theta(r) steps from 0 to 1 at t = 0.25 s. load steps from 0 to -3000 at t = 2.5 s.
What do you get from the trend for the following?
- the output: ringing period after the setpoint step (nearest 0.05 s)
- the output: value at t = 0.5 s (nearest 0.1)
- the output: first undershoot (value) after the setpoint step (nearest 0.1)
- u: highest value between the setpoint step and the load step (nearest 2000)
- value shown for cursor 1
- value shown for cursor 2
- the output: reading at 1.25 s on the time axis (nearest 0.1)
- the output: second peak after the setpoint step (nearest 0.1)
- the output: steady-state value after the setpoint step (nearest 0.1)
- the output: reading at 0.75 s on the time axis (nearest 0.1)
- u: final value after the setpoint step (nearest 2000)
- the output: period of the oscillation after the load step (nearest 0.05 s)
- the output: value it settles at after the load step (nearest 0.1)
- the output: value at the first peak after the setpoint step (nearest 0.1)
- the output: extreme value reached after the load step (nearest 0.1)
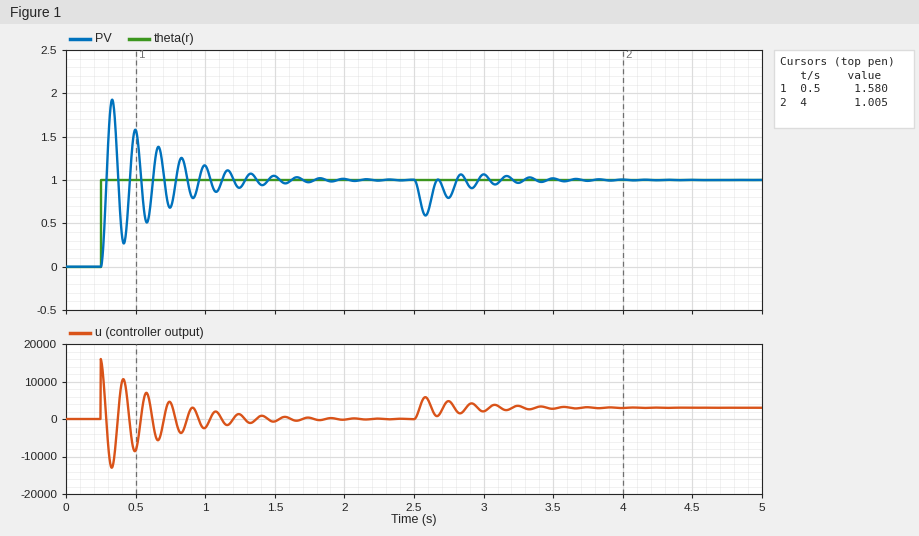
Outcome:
0.15 s
1.6
0.3
16000
1.580
1.005
0.9
1.6
1.0
0.7
0
0.15 s
1.0
1.9
0.6
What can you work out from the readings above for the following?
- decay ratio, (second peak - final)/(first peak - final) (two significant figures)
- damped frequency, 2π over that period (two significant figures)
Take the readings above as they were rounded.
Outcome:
0.67
42 rad/s
